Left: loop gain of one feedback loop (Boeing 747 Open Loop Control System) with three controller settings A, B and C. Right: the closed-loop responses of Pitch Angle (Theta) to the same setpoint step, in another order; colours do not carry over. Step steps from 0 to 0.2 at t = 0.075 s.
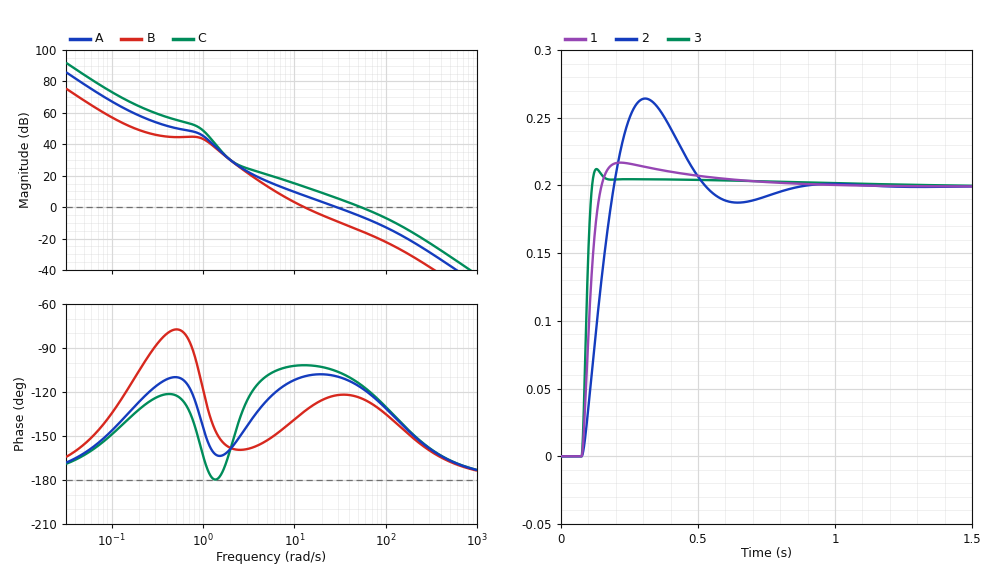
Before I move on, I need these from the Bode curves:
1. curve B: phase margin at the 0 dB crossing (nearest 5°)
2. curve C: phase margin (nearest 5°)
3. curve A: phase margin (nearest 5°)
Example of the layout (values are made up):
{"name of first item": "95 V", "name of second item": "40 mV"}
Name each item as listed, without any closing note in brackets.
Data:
{"curve B: phase margin at the 0 dB crossing": "45°", "curve C: phase margin": "65°", "curve A: phase margin": "70°"}
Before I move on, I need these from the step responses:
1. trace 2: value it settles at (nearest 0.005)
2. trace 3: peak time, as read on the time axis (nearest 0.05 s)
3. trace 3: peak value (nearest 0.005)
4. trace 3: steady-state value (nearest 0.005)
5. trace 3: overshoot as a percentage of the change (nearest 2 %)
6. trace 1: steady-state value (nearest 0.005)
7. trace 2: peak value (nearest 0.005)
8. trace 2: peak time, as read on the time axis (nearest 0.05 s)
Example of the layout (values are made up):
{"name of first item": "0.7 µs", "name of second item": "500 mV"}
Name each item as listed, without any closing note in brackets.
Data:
{"trace 2: value it settles at": "0.200", "trace 3: peak time, as read on the time axis": "0.15 s", "trace 3: peak value": "0.210", "trace 3: steady-state value": "0.200", "trace 3: overshoot as a percentage of the change": "6 %", "trace 1: steady-state value": "0.200", "trace 2: peak value": "0.265", "trace 2: peak time, as read on the time axis": "0.30 s"}
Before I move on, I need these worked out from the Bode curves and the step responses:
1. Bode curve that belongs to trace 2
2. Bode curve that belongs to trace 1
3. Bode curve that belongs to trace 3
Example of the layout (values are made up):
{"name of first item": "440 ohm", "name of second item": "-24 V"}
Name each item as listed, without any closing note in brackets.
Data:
{"Bode curve that belongs to trace 2": "B", "Bode curve that belongs to trace 1": "A", "Bode curve that belongs to trace 3": "C"}
